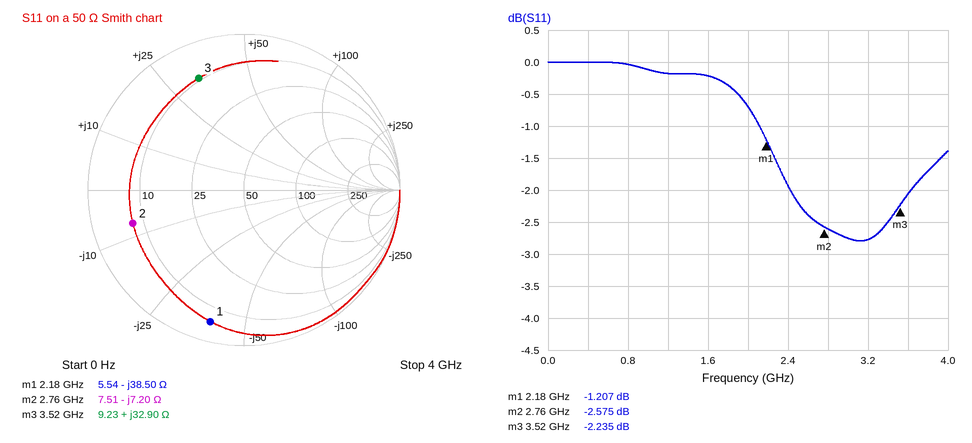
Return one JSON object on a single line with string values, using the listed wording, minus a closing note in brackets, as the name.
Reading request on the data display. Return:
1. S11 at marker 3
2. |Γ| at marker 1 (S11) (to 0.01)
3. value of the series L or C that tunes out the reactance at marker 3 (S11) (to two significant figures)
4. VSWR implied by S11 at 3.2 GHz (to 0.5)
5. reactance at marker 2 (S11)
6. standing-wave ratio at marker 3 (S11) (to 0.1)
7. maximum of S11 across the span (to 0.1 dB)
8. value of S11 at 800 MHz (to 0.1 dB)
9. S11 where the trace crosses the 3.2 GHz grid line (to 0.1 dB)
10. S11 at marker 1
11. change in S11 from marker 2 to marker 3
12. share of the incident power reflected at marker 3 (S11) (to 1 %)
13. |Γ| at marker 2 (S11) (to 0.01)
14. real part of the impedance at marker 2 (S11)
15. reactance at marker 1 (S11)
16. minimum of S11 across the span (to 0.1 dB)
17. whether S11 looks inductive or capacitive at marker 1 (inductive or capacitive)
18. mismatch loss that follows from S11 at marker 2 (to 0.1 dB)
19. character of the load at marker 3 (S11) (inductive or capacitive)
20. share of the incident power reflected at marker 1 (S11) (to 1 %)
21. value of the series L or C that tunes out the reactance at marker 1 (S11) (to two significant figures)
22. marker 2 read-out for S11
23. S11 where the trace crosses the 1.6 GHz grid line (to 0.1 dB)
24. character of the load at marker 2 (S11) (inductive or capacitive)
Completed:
{"S11 at marker 3": "-2.235 dB", "|Γ| at marker 1 (S11)": "0.87", "value of the series L or C that tunes out the reactance at marker 3 (S11)": "1.4 pF", "VSWR implied by S11 at 3.2 GHz": "6.5", "reactance at marker 2": "-7.20 Ω", "standing-wave ratio at marker 3 (S11)": "7.8", "maximum of S11 across the span": "0.0 dB", "value of S11 at 800 MHz": "0.0 dB", "S11 where the trace crosses the 3.2 GHz grid line": "-2.8 dB", "S11 at marker 1": "-1.207 dB", "change in S11 from marker 2 to marker 3": "0.340 dB", "share of the incident power reflected at marker 3 (S11)": "60 %", "|Γ| at marker 2 (S11)": "0.74", "real part of the impedance at marker 2": "7.51 Ω", "reactance at marker 1": "-38.50 Ω", "minimum of S11 across the span": "-2.8 dB", "whether S11 looks inductive or capacitive at marker 1": "capacitive", "mismatch loss that follows from S11 at marker 2": "3.5 dB", "character of the load at marker 3 (S11)": "inductive", "share of the incident power reflected at marker 1 (S11)": "76 %", "value of the series L or C that tunes out the reactance at marker 1 (S11)": "2.8 nH", "marker 2 read-out for S11": "-2.575 dB", "S11 where the trace crosses the 1.6 GHz grid line": "-0.2 dB", "character of the load at marker 2 (S11)": "capacitive"}
